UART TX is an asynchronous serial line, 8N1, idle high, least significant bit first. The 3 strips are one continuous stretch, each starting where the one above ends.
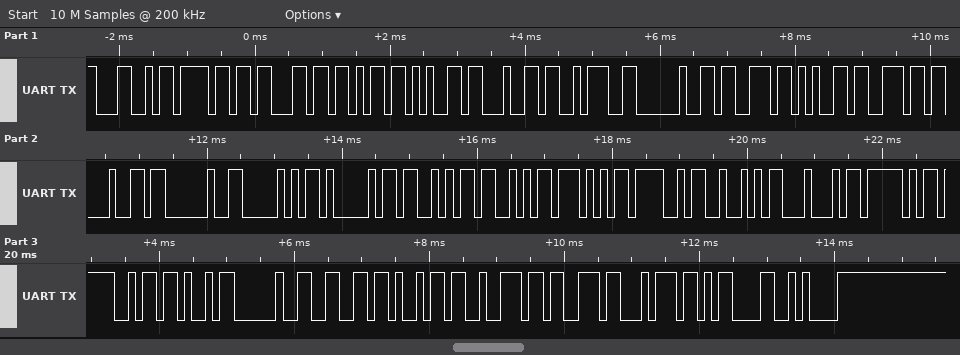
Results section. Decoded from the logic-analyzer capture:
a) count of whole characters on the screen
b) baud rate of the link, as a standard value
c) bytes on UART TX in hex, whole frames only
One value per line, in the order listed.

32
9600 baud
4C 6F 63 6B 65 64 3A 20 73 65 6E 64 20 50 41 53 53 57 4F 52 44 5F 4F 4B 20 66 69 72 73 74 0D 0A
